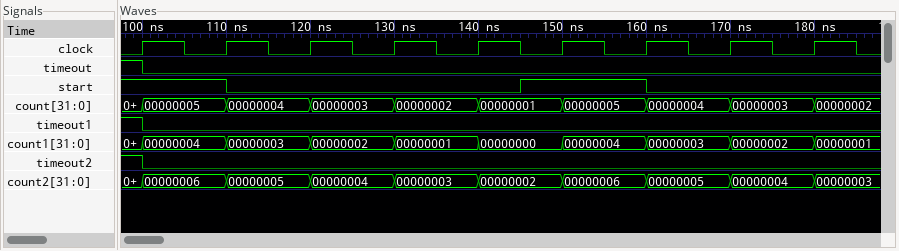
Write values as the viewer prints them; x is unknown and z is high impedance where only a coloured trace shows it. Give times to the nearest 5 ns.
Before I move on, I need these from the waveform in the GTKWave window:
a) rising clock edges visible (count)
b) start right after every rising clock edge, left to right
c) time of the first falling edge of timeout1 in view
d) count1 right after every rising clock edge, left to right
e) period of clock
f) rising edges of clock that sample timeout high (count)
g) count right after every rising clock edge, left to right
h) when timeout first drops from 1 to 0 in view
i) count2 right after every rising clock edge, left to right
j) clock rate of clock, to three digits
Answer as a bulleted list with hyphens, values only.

- 9
- 1 0 0 0 0 1 0 0 0
- 100 ns
- 00000004, 00000003, 00000002, 00000001, 00000000, 00000004, 00000003, 00000002, 00000001
- 10 ns
- 1
- 00000005, 00000004, 00000003, 00000002, 00000001, 00000005, 00000004, 00000003, 00000002
- 100 ns
- 00000006, 00000005, 00000004, 00000003, 00000002, 00000006, 00000005, 00000004, 00000003
- 100 MHz
